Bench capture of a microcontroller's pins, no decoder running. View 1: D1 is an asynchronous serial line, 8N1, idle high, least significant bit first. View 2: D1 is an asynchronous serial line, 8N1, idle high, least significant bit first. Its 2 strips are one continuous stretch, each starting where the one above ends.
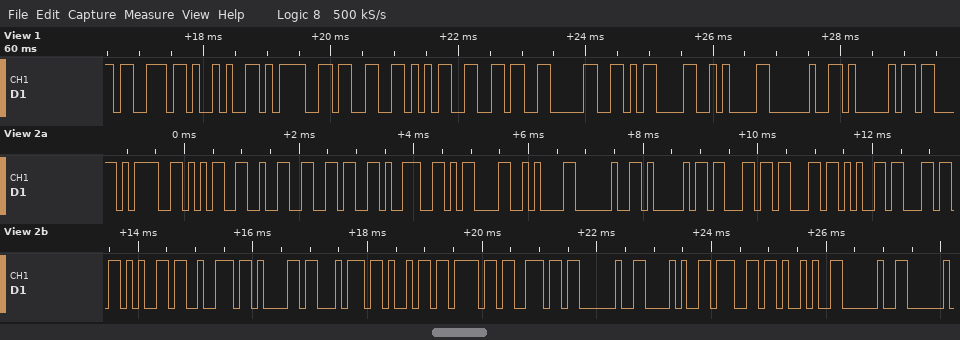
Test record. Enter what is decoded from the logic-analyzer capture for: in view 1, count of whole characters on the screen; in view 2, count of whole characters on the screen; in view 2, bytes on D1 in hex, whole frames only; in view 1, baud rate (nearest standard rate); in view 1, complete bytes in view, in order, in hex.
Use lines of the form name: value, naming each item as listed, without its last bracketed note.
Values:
in view 1, count of whole characters on the screen: 11
in view 2, count of whole characters on the screen: 25
in view 2, bytes on D1 in hex, whole frames only: 3D 35 32 36 39 0D 0A 20 41 63 63 65 6C 65 72 61 74 69 6F 6E 20 28 67 29 20
in view 1, baud rate: 9600 baud
in view 1, complete bytes in view, in order, in hex: 73 29 3D 33 35 36 30 0D 0A 20 41
